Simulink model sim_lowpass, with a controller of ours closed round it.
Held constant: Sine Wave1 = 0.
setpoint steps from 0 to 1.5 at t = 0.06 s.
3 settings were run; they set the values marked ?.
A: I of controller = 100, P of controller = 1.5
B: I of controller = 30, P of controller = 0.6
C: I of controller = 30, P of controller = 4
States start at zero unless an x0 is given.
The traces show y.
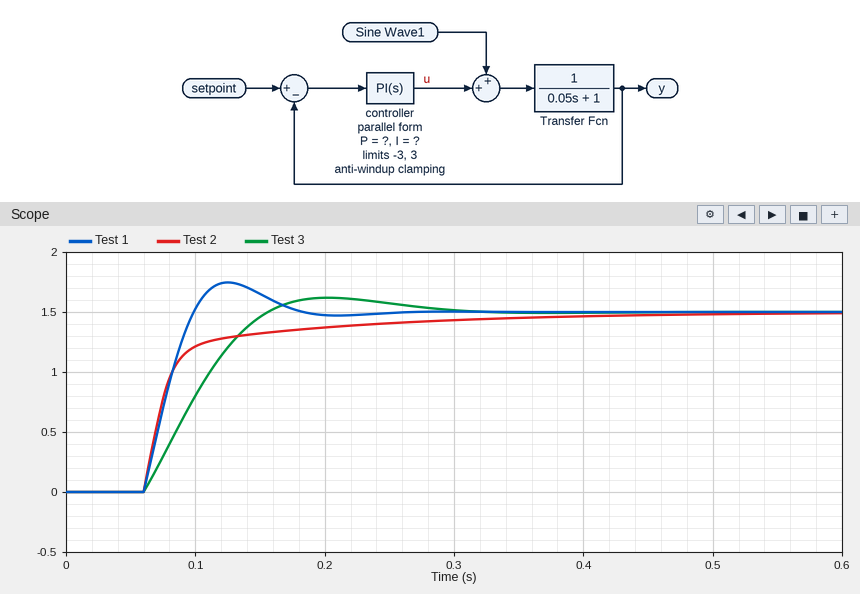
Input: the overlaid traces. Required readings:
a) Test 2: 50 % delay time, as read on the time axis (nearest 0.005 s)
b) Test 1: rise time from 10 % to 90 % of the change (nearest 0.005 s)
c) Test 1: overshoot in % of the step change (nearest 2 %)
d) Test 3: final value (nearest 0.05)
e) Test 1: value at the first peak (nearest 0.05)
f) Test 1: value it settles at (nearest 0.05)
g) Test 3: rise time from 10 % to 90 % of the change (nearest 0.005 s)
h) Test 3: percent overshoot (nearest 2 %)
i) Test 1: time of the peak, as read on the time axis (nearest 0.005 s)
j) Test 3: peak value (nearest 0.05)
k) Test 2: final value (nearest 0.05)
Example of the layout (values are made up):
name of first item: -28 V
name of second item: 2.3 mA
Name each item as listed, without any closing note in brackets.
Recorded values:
Test 2: 50 % delay time, as read on the time axis: 0.075 s
Test 1: rise time from 10 % to 90 % of the change: 0.030 s
Test 1: overshoot in % of the step change: 16 %
Test 3: final value: 1.50
Test 1: value at the first peak: 1.75
Test 1: value it settles at: 1.50
Test 3: rise time from 10 % to 90 % of the change: 0.070 s
Test 3: percent overshoot: 8 %
Test 1: time of the peak, as read on the time axis: 0.125 s
Test 3: peak value: 1.60
Test 2: final value: 1.50
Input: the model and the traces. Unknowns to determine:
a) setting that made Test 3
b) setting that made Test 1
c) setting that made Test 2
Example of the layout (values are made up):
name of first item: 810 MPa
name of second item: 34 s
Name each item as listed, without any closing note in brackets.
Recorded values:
setting that made Test 3: B
setting that made Test 1: A
setting that made Test 2: C
